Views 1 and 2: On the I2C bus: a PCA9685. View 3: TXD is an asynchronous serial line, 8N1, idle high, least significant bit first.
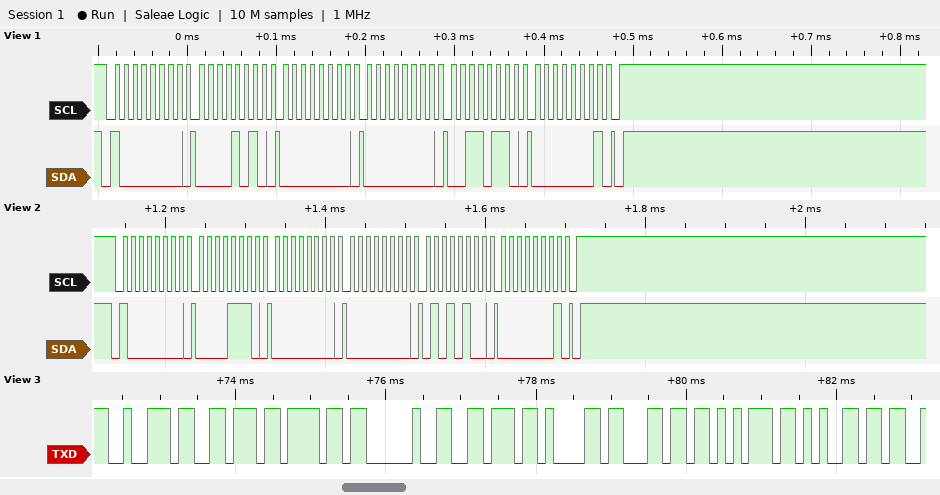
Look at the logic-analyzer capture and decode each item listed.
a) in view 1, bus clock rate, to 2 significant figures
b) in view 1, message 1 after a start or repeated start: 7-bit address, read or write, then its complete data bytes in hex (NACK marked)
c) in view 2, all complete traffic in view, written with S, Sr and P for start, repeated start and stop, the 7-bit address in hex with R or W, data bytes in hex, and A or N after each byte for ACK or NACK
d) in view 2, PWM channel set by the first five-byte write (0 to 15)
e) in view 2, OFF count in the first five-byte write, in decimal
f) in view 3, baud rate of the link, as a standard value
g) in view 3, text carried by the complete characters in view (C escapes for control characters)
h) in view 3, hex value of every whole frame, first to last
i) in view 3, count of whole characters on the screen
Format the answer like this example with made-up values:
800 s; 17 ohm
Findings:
100 kHz; 0x40 write: 0A 00 00 36 01; S 40W A 0E A 00 A 00 A 54 A 01 A P; 2; 340; 9600 baud; "rvo value"; 72 76 6F 20 76 61 6C 75 65; 9
